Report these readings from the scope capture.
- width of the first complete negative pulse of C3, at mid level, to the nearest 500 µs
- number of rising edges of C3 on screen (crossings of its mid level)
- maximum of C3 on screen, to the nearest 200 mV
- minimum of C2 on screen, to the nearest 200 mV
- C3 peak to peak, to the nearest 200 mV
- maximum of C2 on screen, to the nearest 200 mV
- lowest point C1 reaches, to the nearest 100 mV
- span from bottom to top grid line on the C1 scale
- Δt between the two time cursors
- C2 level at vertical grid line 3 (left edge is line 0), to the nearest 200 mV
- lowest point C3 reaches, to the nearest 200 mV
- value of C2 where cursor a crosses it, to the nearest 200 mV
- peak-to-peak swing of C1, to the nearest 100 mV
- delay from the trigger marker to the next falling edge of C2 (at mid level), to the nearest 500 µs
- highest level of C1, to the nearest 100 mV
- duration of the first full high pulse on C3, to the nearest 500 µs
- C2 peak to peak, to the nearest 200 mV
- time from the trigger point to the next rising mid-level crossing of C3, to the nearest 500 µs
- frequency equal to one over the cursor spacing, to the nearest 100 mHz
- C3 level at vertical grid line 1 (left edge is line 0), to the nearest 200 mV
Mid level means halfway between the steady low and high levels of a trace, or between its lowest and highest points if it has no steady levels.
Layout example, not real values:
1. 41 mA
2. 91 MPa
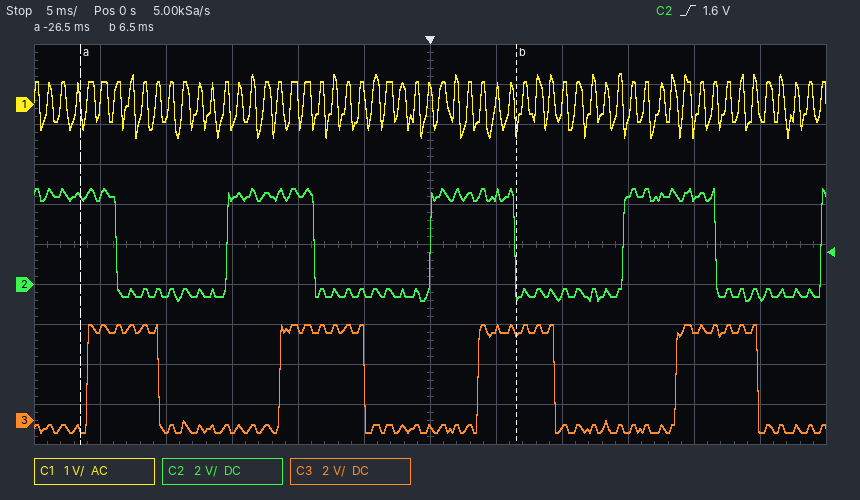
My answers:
1. 9.0 ms
2. 4
3. 4.8 V
4. -800 mV
5. 5.4 V
6. 4.8 V
7. -800 mV
8. 10 V
9. 33.0 ms
10. 4.4 V
11. -600 mV
12. 4.4 V
13. 1.6 V
14. 6.5 ms
15. 800 mV
16. 5.5 ms
17. 5.6 V
18. 3.5 ms
19. 30.3 Hz
20. 4.6 V
